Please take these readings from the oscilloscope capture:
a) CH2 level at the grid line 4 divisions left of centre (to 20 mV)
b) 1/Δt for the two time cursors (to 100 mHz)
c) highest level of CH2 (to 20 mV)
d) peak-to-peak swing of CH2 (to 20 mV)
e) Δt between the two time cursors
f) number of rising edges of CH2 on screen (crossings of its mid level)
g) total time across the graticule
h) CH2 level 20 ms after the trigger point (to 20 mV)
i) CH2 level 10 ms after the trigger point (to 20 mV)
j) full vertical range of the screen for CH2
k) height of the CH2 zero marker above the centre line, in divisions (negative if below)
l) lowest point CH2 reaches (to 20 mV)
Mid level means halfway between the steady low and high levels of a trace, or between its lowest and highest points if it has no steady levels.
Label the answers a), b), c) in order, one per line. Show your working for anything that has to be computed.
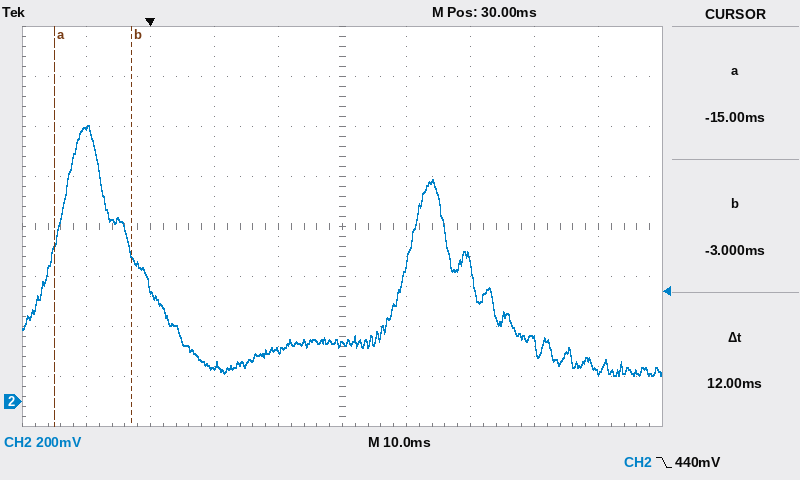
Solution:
a) 1.10 V
b) 1 / 12 ms ≈ 83.3 Hz
c) 1.10 V
d) 1.10 V − (100 mV) = 1.00 V
e) 12 ms
f) 2
g) 100 ms
h) 200 mV
i) 140 mV
j) 1.6 V
k) -3.5 div
l) 100 mV
